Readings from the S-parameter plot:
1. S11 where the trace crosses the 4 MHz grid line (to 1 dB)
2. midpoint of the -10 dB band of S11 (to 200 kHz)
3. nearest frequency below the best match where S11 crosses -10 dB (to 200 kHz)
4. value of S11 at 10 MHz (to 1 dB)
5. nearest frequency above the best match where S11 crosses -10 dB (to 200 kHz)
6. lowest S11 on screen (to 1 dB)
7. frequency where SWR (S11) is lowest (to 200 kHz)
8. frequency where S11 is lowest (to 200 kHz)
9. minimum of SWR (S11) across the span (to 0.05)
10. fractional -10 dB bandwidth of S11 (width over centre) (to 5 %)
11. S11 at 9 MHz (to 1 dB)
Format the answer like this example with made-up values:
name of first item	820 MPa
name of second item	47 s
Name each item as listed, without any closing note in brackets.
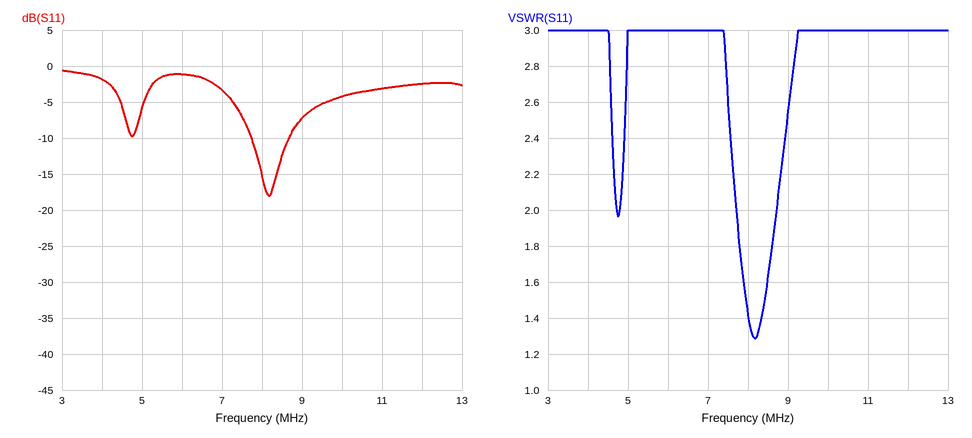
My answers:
S11 where the trace crosses the 4 MHz grid line	-2 dB
midpoint of the -10 dB band of S11	8.2 MHz
nearest frequency below the best match where S11 crosses -10 dB	7.8 MHz
value of S11 at 10 MHz	-4 dB
nearest frequency above the best match where S11 crosses -10 dB	8.6 MHz
lowest S11 on screen	-18 dB
frequency where SWR (S11) is lowest	8.2 MHz
frequency where S11 is lowest	8.2 MHz
minimum of SWR (S11) across the span	1.30
fractional -10 dB bandwidth of S11 (width over centre)	10 %
S11 at 9 MHz	-7 dB
